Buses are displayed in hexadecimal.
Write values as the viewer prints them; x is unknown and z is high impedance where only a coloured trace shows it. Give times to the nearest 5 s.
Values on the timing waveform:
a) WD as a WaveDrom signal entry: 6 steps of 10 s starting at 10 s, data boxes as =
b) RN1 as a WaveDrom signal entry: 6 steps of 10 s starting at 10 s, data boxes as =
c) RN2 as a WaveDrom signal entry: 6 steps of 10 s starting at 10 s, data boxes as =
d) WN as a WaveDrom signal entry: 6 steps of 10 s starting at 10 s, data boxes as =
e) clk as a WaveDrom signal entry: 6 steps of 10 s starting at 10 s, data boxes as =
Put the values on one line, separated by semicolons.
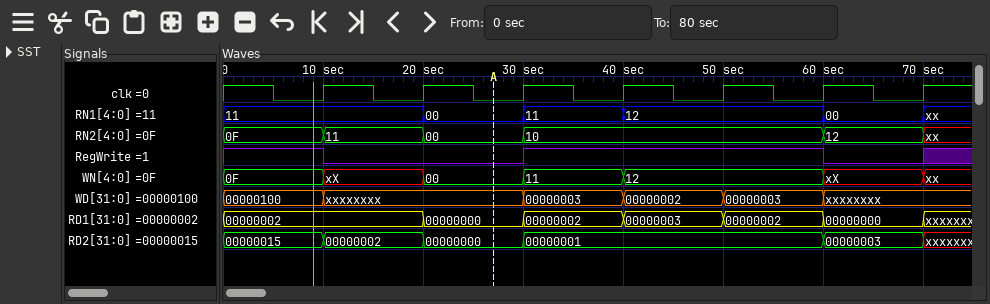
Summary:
{name: 'WD', wave: 'x.===x', data: '00000003 00000002 00000003'}; {name: 'RN1', wave: '====.=', data: '11 00 11 12 00'}; {name: 'RN2', wave: '===..=', data: '11 00 10 12'}; {name: 'WN', wave: '====.=', data: 'xX 00 11 12 xX'}; {name: 'clk', wave: 'p.....'}
